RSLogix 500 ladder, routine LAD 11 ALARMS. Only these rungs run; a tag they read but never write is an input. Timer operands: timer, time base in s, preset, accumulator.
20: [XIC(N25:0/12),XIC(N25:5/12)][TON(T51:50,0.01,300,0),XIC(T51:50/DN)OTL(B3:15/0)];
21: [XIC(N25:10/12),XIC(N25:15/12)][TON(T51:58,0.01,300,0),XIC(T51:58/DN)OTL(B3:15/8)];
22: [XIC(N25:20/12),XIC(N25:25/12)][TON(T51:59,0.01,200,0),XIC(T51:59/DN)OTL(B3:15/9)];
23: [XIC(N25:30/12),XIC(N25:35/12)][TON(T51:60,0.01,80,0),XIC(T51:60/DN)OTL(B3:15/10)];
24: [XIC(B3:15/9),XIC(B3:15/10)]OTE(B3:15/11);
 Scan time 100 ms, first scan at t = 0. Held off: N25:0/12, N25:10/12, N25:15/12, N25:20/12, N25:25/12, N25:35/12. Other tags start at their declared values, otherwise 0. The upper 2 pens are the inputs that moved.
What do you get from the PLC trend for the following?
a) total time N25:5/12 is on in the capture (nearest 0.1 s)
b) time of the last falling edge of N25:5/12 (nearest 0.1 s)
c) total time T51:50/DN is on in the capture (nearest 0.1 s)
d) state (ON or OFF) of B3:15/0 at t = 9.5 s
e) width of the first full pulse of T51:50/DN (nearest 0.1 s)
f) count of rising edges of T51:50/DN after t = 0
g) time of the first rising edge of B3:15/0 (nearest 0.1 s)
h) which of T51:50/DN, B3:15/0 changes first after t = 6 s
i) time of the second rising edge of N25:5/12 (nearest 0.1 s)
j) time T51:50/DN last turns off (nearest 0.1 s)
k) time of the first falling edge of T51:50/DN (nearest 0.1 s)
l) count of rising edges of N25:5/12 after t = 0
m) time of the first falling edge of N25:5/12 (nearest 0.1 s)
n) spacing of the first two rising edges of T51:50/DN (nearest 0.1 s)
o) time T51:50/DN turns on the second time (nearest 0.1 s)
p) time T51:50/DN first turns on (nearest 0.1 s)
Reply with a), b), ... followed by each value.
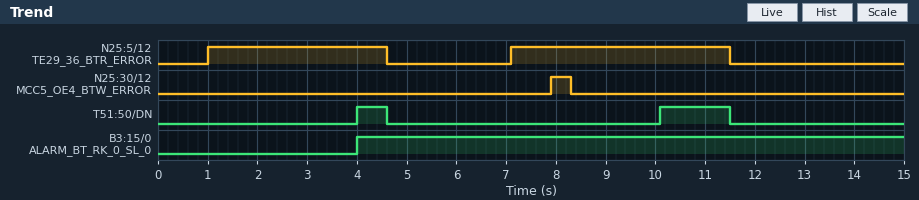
a) 8.0 s
b) 11.5 s
c) 2.0 s
d) ON
e) 0.6 s
f) 2
g) 4.0 s
h) T51:50/DN
i) 7.1 s
j) 11.5 s
k) 4.6 s
l) 2
m) 4.6 s
n) 6.1 s
o) 10.1 s
p) 4.0 s
